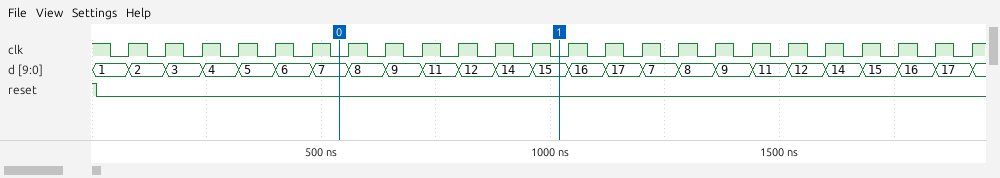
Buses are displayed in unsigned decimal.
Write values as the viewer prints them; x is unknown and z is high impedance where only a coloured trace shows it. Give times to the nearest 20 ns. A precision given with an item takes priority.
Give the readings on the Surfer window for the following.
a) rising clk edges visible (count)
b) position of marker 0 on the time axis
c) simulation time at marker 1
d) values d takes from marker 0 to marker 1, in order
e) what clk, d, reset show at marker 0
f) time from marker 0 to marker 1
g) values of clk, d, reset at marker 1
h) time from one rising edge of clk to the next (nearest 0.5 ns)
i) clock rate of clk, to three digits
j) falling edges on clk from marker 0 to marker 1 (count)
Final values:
24
540 ns
1020 ns
7, 8, 9, 11, 12, 14, 15
clk=0, d=7, reset=0
480 ns
clk=0, d=15, reset=0
80 ns
12.5 MHz
6
